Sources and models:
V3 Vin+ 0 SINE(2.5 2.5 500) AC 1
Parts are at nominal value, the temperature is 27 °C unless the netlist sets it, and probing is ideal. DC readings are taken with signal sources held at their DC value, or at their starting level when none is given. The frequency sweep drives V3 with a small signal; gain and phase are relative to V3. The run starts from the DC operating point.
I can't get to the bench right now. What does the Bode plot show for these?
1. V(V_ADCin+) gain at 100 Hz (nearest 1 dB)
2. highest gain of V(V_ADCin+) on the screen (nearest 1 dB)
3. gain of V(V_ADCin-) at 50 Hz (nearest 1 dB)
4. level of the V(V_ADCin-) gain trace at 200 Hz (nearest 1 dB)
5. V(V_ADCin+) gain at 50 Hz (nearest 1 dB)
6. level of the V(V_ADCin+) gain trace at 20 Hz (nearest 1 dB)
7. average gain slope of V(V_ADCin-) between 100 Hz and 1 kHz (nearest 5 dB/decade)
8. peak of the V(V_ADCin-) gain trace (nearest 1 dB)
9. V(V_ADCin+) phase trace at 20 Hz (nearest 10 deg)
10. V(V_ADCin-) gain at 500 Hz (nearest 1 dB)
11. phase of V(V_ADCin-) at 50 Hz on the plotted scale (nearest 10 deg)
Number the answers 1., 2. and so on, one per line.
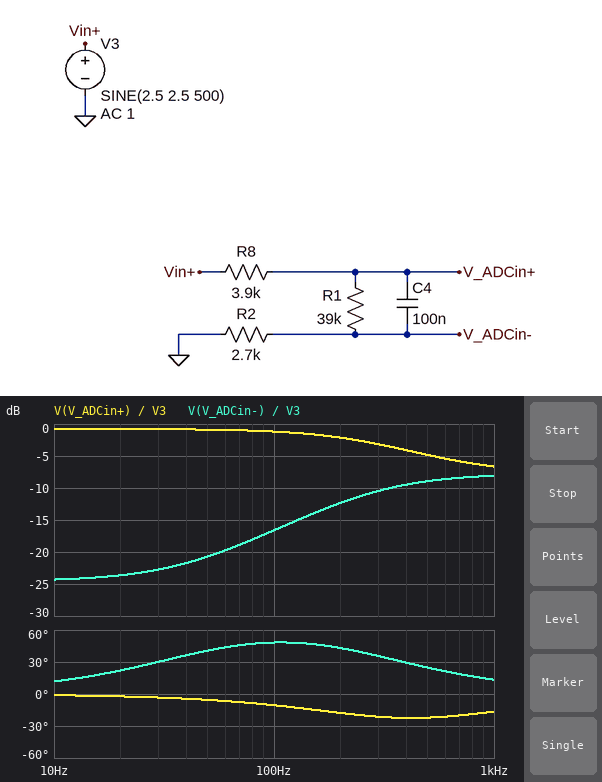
1. -1 dB
2. -1 dB
3. -21 dB
4. -12 dB
5. -1 dB
6. -1 dB
7. 10 dB/decade
8. -8 dB
9. 0 deg
10. -9 dB
11. 40 deg
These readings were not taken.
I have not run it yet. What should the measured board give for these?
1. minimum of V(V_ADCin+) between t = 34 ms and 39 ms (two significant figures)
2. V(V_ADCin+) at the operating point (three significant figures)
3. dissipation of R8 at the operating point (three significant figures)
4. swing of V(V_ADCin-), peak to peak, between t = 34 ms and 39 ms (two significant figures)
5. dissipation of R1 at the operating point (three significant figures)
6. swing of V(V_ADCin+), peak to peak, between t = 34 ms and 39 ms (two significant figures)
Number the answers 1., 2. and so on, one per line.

1. 850 mV
2. 2.29 V
3. 11.7 µW
4. 1.8 V
5. 117 µW
6. 2.9 V
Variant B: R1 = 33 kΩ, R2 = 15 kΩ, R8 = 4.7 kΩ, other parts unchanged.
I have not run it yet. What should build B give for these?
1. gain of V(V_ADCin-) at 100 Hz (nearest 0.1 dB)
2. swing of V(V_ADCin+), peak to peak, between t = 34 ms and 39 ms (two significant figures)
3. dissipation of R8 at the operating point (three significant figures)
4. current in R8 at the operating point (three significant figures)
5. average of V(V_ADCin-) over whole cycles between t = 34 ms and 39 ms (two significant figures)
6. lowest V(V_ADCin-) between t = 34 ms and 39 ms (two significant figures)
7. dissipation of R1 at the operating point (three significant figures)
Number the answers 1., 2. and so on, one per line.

1. -5.7 dB
2. 3.9 V
3. 10.6 µW
4. 47.4 µA
5. 710 mV
6. -1.1 V
7. 74.3 µW
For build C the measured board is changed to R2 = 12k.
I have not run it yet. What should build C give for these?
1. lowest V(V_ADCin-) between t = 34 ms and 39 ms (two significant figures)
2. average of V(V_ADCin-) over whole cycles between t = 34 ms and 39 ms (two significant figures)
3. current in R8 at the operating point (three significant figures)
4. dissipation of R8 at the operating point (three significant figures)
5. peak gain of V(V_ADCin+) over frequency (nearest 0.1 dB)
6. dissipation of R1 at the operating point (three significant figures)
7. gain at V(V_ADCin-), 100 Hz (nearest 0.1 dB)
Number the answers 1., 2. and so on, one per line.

1. -1.3 V
2. 550 mV
3. 45.5 µA
4. 8.09 µW
5. -0.6 dB
6. 80.9 µW
7. -6.5 dB
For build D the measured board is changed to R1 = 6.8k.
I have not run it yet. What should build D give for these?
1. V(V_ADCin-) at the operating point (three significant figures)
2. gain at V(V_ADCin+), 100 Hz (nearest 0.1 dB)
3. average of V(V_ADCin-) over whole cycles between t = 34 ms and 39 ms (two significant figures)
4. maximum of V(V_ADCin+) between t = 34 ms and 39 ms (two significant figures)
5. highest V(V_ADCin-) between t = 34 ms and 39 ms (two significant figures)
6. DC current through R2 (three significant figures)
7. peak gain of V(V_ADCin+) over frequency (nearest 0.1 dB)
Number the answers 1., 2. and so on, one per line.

1. 504 mV
2. -3.1 dB
3. 500 mV
4. 3.2 V
5. 1.3 V
6. 187 µA
7. -3.0 dB
